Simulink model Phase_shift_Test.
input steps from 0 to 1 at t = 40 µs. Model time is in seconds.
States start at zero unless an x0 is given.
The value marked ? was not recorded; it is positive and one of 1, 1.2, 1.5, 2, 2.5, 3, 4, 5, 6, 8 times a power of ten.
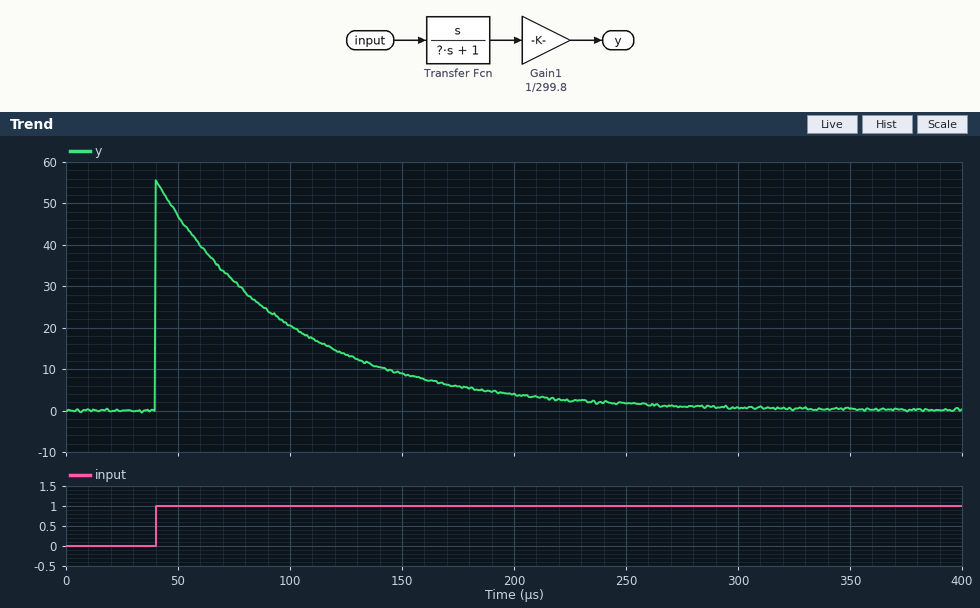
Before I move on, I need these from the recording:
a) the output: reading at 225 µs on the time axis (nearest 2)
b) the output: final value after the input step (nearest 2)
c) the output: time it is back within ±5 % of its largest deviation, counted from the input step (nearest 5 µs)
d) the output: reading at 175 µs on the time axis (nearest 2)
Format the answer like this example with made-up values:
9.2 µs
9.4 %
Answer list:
2
0
180 µs
6
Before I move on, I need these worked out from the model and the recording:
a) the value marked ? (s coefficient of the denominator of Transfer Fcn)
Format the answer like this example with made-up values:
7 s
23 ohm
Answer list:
6e-05
